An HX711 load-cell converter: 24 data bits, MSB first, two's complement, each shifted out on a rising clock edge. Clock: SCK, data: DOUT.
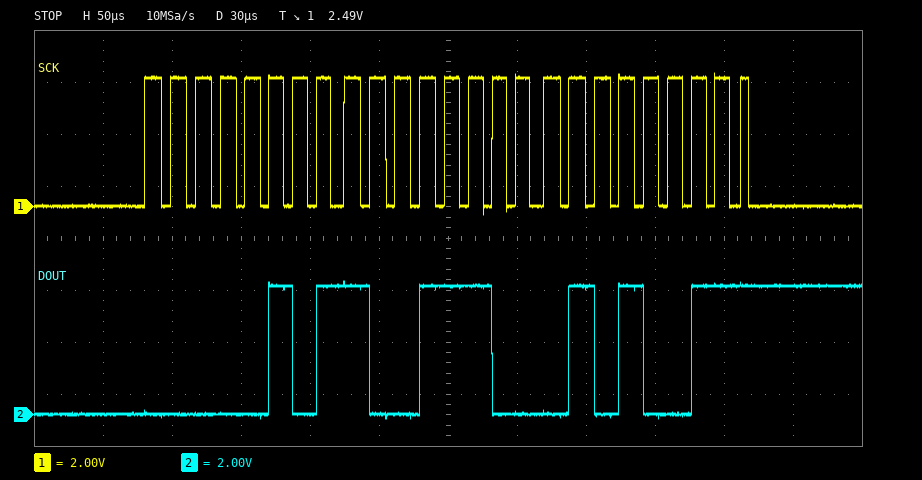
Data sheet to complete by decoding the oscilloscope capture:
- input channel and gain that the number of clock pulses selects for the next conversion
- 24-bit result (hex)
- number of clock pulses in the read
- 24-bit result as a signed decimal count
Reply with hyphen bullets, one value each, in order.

- channel A, gain 128
- 0x059C53
- 25
- 367699
